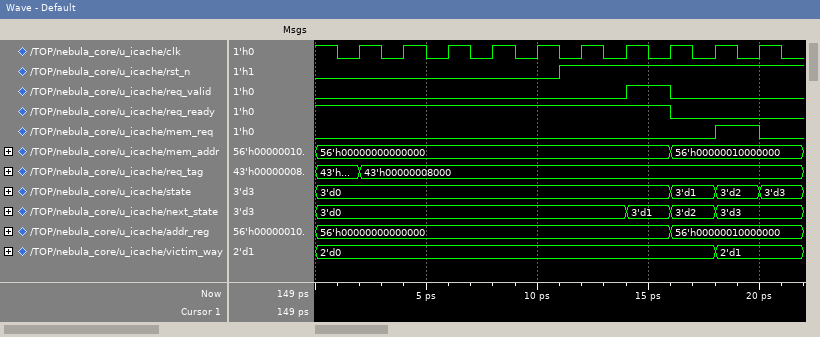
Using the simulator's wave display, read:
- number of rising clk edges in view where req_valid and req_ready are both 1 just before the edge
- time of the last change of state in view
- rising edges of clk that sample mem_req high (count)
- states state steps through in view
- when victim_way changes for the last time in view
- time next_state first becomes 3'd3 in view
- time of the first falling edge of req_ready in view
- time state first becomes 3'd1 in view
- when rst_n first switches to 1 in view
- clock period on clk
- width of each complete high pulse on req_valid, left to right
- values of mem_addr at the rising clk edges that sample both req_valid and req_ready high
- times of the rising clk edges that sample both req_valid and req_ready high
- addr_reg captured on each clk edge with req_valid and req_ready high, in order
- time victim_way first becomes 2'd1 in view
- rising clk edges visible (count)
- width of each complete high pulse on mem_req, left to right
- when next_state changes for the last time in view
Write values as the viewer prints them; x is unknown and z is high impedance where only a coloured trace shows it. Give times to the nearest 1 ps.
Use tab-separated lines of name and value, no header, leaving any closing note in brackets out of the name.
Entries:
number of rising clk edges in view where req_valid and req_ready are both 1 just before the edge	1
time of the last change of state in view	20 ps
rising edges of clk that sample mem_req high	1
states state steps through in view	3'd0, 3'd1, 3'd2, 3'd3
when victim_way changes for the last time in view	18 ps
time next_state first becomes 3'd3 in view	18 ps
time of the first falling edge of req_ready in view	16 ps
time state first becomes 3'd1 in view	16 ps
when rst_n first switches to 1 in view	11 ps
clock period on clk	2 ps
width of each complete high pulse on req_valid, left to right	2 ps
values of mem_addr at the rising clk edges that sample both req_valid and req_ready high	56'h00000000000000
times of the rising clk edges that sample both req_valid and req_ready high	16 ps
addr_reg captured on each clk edge with req_valid and req_ready high, in order	56'h00000000000000
time victim_way first becomes 2'd1 in view	18 ps
rising clk edges visible	10
width of each complete high pulse on mem_req, left to right	2 ps
when next_state changes for the last time in view	18 ps
